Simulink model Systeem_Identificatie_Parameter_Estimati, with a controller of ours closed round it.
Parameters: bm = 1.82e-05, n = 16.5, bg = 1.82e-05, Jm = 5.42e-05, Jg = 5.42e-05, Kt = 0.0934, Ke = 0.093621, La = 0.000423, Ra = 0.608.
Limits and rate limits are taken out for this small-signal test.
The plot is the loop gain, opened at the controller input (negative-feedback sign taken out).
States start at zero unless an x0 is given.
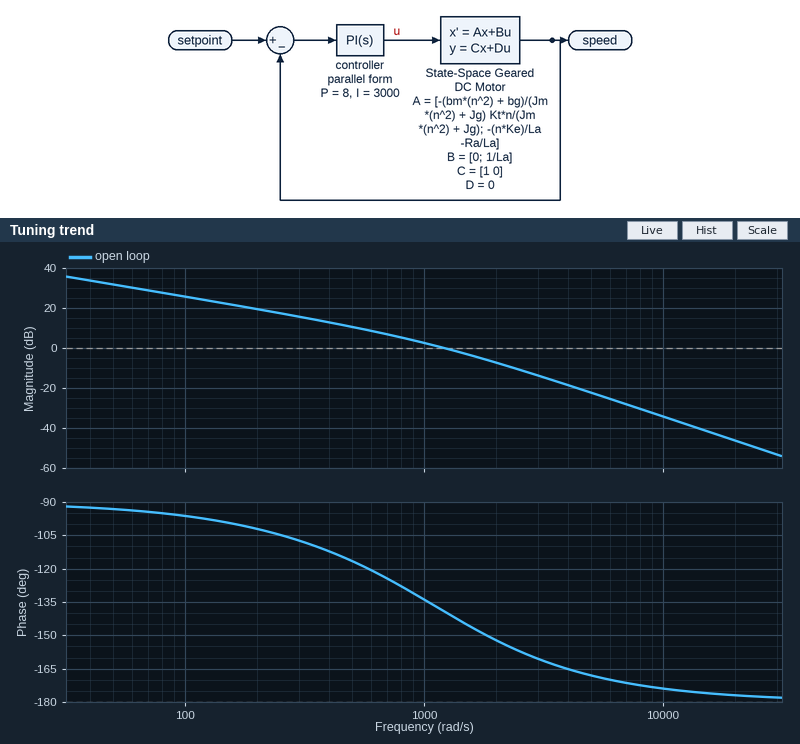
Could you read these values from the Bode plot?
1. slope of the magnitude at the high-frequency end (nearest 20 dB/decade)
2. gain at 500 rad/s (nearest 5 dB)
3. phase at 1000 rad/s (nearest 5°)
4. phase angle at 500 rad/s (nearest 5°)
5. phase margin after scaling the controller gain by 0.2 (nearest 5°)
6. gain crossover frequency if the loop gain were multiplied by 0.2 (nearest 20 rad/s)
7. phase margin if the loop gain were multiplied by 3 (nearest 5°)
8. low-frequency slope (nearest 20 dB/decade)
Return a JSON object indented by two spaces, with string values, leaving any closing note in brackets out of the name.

{
  "slope of the magnitude at the high-frequency end": "-40 dB/decade",
  "gain at 500 rad/s": "10 dB",
  "phase at 1000 rad/s": "-135°",
  "phase angle at 500 rad/s": "-115°",
  "phase margin after scaling the controller gain by 0.2": "70°",
  "gain crossover frequency if the loop gain were multiplied by 0.2": "360 rad/s",
  "phase margin if the loop gain were multiplied by 3": "25°",
  "low-frequency slope": "-20 dB/decade"
}
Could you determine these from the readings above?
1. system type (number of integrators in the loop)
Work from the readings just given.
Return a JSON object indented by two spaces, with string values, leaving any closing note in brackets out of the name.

{
  "system type": "1"
}
